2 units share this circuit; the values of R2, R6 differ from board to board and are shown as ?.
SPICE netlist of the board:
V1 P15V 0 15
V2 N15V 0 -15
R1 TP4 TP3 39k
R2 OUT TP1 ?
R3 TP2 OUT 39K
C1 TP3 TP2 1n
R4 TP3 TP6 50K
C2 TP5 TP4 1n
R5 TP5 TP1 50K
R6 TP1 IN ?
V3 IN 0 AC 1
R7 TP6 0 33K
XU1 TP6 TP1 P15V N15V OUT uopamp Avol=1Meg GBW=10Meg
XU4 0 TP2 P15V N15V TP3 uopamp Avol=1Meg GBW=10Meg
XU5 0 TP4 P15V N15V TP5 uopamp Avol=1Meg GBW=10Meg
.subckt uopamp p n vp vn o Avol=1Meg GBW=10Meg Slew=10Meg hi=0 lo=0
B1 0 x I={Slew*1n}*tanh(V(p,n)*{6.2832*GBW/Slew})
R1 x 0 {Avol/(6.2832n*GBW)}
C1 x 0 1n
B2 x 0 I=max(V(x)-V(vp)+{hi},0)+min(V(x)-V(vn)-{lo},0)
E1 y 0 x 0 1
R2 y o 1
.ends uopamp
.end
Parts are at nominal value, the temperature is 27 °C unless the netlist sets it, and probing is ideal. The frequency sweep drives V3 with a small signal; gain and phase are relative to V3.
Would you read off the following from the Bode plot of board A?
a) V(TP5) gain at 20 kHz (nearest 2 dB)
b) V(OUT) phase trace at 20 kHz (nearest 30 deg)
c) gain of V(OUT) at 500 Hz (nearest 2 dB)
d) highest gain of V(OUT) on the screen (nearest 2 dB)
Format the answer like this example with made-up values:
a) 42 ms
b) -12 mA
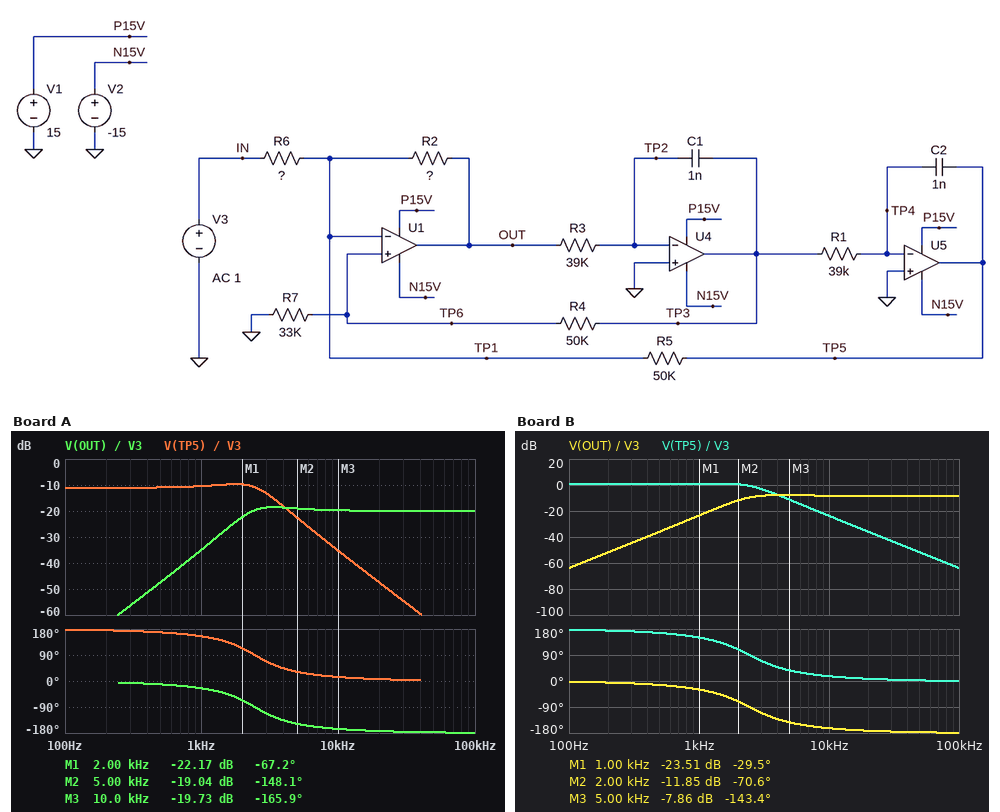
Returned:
a) -48 dB
b) -180 deg
c) -48 dB
d) -18 dB
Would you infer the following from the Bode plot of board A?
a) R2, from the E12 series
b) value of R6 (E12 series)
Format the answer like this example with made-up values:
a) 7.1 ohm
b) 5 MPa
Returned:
a) 18 kΩ
b) 180 kΩ
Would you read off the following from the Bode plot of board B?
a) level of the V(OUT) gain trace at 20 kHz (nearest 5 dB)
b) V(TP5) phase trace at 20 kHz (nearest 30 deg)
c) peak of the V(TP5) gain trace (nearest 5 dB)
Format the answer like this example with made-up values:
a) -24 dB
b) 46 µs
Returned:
a) -10 dB
b) 0 deg
c) 0 dB
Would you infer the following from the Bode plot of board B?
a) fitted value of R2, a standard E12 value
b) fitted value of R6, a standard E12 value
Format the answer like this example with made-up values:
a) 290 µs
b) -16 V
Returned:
a) 18 kΩ
b) 47 kΩ
